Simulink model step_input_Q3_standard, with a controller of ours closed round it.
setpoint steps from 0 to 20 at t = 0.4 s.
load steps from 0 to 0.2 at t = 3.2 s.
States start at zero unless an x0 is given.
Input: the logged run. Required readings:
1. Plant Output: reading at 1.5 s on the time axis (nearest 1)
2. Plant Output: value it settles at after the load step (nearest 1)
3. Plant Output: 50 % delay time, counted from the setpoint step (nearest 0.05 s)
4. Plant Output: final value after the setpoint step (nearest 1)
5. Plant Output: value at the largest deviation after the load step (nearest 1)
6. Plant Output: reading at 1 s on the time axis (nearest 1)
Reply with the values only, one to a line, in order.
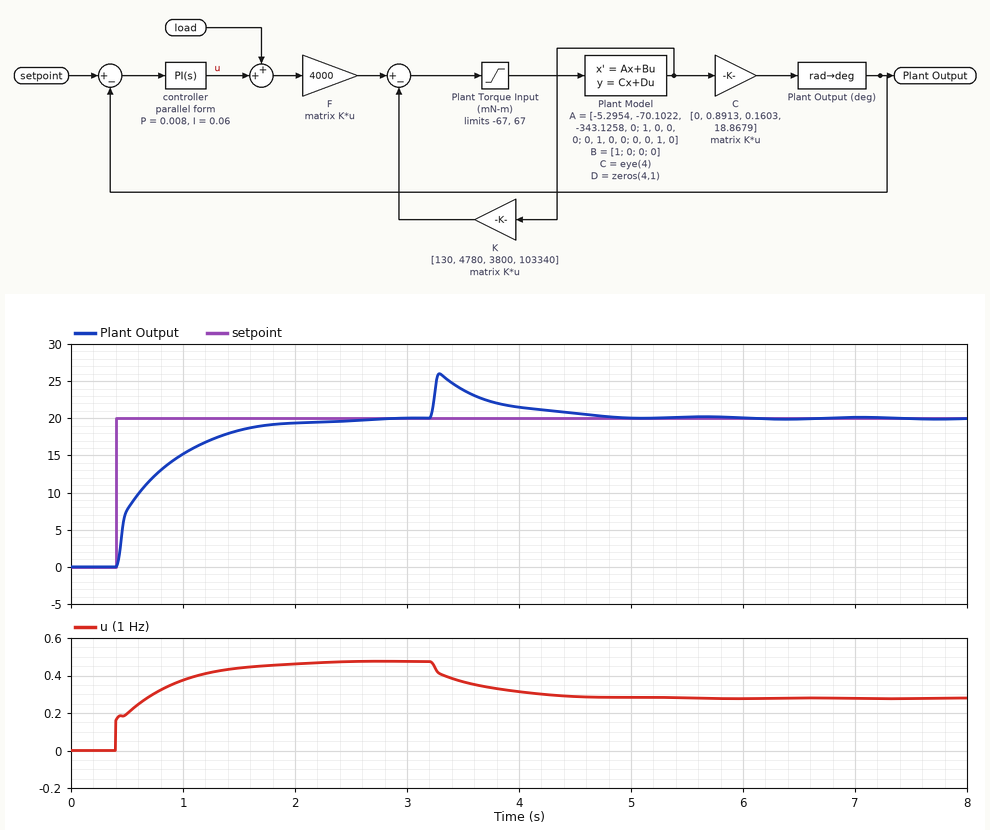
18
20
0.20 s
20
26
15
